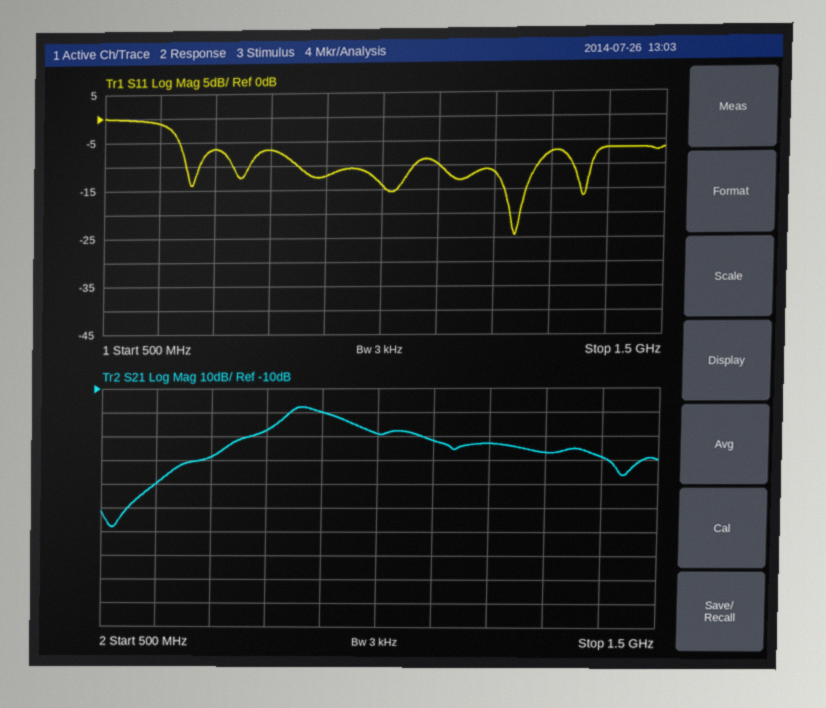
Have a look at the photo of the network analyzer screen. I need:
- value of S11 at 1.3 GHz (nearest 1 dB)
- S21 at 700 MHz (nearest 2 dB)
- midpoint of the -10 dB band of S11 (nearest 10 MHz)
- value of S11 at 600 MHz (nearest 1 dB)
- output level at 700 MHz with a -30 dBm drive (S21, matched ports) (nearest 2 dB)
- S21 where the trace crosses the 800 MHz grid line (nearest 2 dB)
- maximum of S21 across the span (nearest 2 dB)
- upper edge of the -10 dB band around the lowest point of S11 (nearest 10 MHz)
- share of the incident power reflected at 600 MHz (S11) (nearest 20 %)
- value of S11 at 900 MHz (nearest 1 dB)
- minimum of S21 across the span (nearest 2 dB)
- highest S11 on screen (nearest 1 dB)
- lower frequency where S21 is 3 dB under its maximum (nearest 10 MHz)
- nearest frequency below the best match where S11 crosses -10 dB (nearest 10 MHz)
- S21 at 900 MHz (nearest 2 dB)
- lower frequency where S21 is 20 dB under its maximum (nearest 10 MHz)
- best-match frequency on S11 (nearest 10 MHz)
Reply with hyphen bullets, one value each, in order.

- -7 dB
- -38 dB
- 1.19 GHz
- -1 dB
- -68 dBm
- -28 dB
- -18 dB
- 1.28 GHz
- 80 %
- -12 dB
- -68 dB
- 0 dB
- 840 MHz
- 1.10 GHz
- -20 dB
- 710 MHz
- 1.24 GHz
